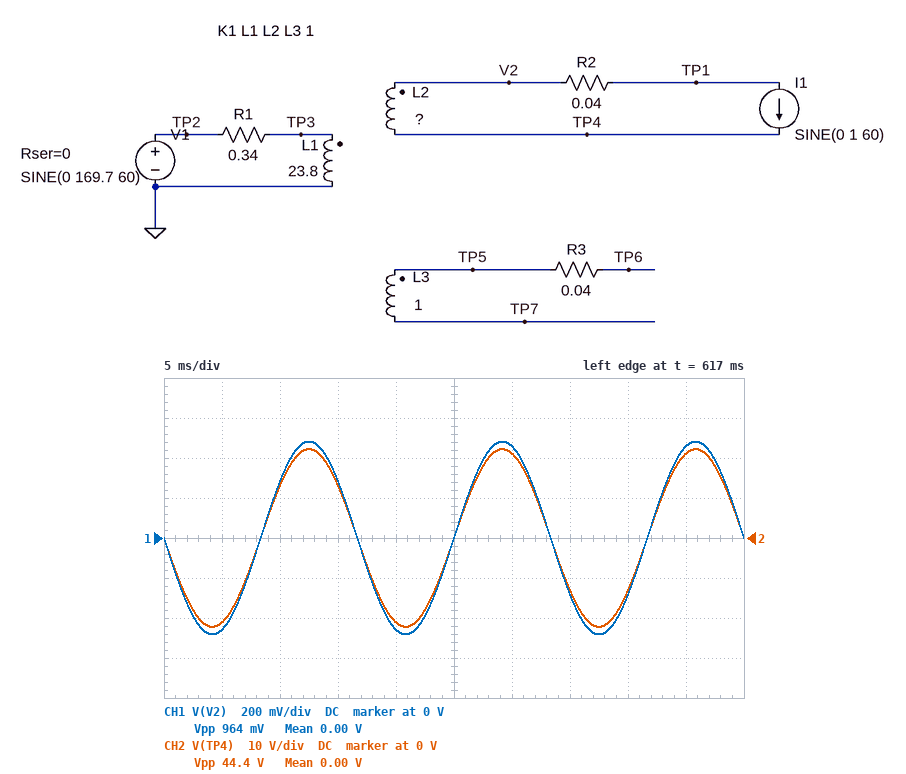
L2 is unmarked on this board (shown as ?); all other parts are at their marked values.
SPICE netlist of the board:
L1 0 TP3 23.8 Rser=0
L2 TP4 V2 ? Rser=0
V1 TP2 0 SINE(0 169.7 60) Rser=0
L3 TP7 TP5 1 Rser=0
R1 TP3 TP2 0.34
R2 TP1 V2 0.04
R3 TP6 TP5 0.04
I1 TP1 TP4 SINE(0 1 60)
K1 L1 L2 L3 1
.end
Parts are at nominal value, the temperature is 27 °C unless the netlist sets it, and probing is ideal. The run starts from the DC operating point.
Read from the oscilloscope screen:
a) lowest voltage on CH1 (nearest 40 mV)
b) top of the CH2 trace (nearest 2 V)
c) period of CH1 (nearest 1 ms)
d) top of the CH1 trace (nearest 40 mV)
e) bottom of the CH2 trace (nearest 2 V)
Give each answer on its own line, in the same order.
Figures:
-480 mV
22 V
17 ms
480 mV
-22 V
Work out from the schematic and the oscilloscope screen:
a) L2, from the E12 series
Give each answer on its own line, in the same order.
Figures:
390 mH
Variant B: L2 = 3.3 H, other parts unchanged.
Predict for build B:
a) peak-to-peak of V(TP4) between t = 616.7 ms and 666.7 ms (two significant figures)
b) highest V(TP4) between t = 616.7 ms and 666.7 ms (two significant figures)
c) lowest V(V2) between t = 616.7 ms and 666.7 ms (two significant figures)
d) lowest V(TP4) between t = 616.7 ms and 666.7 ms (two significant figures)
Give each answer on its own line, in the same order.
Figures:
130 V
64 V
-480 mV
-64 V
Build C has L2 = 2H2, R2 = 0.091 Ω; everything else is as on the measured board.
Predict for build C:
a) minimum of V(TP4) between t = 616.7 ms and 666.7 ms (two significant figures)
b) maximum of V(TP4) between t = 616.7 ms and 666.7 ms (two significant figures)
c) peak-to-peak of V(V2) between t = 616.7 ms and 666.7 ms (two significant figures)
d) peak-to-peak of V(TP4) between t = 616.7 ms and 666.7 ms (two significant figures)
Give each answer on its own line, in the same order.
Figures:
-52 V
52 V
910 mV
100 V
